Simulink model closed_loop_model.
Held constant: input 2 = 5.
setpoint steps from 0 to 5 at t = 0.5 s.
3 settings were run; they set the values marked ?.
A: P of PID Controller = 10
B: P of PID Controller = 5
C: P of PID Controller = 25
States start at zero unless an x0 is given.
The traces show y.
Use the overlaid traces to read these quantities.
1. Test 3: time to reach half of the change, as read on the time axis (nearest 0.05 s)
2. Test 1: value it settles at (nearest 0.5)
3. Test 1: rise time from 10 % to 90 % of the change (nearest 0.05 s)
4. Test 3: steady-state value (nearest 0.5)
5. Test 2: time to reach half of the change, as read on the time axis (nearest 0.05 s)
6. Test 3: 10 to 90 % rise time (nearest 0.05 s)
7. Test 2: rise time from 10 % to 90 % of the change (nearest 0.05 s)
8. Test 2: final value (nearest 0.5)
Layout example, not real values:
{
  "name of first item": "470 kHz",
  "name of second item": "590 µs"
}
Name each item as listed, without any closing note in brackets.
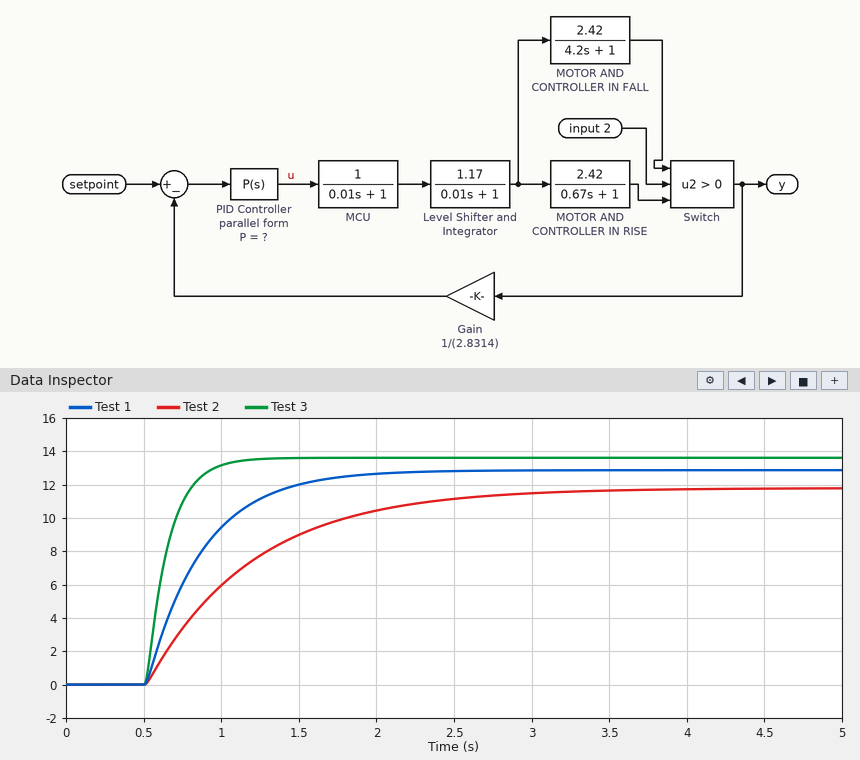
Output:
{
  "Test 3: time to reach half of the change, as read on the time axis": "0.60 s",
  "Test 1: value it settles at": "13.0",
  "Test 1: rise time from 10 % to 90 % of the change": "0.80 s",
  "Test 3: steady-state value": "13.5",
  "Test 2: time to reach half of the change, as read on the time axis": "1.00 s",
  "Test 3: 10 to 90 % rise time": "0.30 s",
  "Test 2: rise time from 10 % to 90 % of the change": "1.50 s",
  "Test 2: final value": "12.0"
}
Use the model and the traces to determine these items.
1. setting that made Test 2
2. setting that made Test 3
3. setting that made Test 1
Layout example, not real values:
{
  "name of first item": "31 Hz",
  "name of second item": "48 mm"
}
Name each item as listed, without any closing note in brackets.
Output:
{
  "setting that made Test 2": "B",
  "setting that made Test 3": "C",
  "setting that made Test 1": "A"
}
